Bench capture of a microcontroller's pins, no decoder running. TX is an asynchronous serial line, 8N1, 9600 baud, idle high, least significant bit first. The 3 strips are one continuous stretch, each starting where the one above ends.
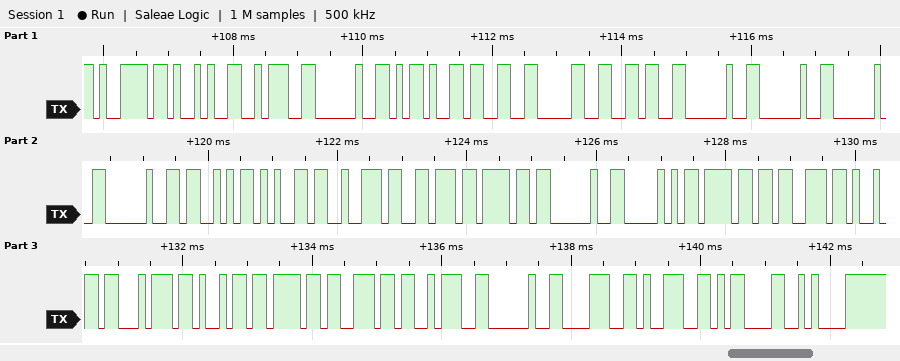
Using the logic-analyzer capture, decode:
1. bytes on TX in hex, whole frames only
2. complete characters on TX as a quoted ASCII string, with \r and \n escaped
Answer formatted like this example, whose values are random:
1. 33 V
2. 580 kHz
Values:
1. 0x79 0x29 0x3A 0x20 0x2D 0x33 0x30 0x36 0x20 0x20 0x20 0x20 0x53 0x65 0x72 0x76 0x6F 0x20 0x50 0x6F 0x73 0x69 0x74 0x69 0x6F 0x6E 0x3A 0x20 0x38 0x39 0x0D 0x0A
2. "y): -306    Servo Position: 89\r\n"
